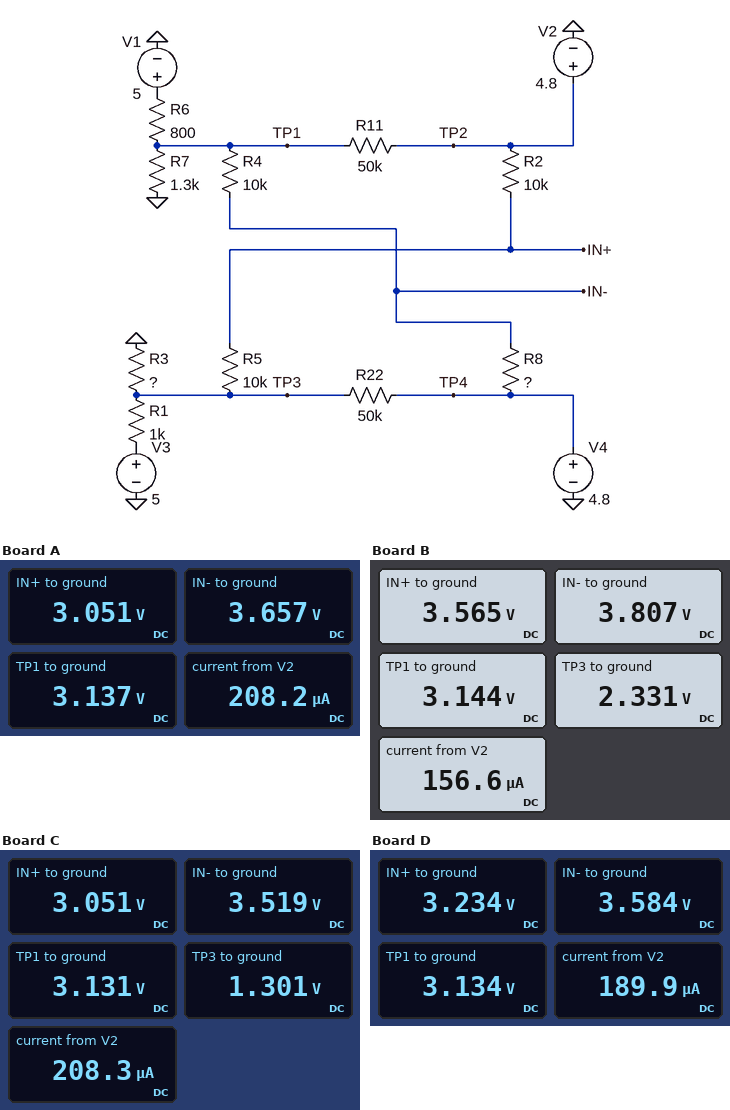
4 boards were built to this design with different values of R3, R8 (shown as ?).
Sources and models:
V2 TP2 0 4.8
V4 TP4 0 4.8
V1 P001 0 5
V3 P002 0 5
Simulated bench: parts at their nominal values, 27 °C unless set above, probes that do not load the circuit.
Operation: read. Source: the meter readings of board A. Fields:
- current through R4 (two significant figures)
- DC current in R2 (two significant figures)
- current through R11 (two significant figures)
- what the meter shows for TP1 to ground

52 µA
170 µA
33 µA
3.137 V
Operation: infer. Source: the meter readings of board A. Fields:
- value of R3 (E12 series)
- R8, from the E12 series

330 Ω
22 kΩ
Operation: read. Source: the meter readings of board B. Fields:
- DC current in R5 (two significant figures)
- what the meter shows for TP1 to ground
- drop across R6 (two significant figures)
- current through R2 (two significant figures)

120 µA
3.144 V
1.9 V
120 µA
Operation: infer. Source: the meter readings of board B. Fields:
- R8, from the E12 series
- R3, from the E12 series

15 kΩ
820 Ω
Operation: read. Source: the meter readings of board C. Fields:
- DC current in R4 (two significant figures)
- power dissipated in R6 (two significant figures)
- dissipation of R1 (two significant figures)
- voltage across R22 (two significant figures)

39 µA
4.4 mW
14 mW
3.5 V
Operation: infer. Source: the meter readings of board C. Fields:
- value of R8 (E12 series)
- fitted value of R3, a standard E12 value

33 kΩ
330 Ω
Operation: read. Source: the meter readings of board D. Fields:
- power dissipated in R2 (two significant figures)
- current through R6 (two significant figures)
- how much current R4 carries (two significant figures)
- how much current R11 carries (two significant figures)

250 µW
2.3 mA
45 µA
33 µA
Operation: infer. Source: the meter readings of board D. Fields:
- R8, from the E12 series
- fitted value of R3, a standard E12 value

27 kΩ
470 Ω
